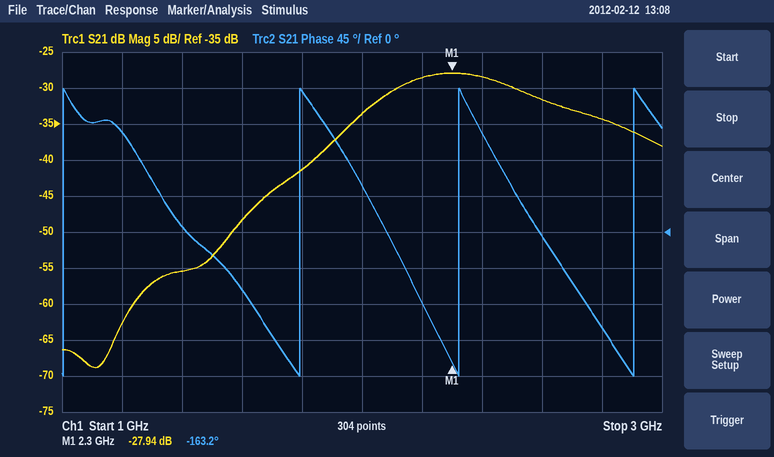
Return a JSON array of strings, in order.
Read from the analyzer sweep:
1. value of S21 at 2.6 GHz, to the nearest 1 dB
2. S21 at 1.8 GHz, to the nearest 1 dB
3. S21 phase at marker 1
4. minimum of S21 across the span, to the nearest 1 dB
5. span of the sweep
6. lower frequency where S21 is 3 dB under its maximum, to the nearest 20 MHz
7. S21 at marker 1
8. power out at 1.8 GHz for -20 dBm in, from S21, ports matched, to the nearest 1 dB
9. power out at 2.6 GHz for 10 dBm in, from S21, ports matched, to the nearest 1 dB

["-32 dB", "-41 dB", "-163.2°", "-69 dB", "2 GHz", "2.08 GHz", "-27.94 dB", "-61 dBm", "-22 dBm"]
